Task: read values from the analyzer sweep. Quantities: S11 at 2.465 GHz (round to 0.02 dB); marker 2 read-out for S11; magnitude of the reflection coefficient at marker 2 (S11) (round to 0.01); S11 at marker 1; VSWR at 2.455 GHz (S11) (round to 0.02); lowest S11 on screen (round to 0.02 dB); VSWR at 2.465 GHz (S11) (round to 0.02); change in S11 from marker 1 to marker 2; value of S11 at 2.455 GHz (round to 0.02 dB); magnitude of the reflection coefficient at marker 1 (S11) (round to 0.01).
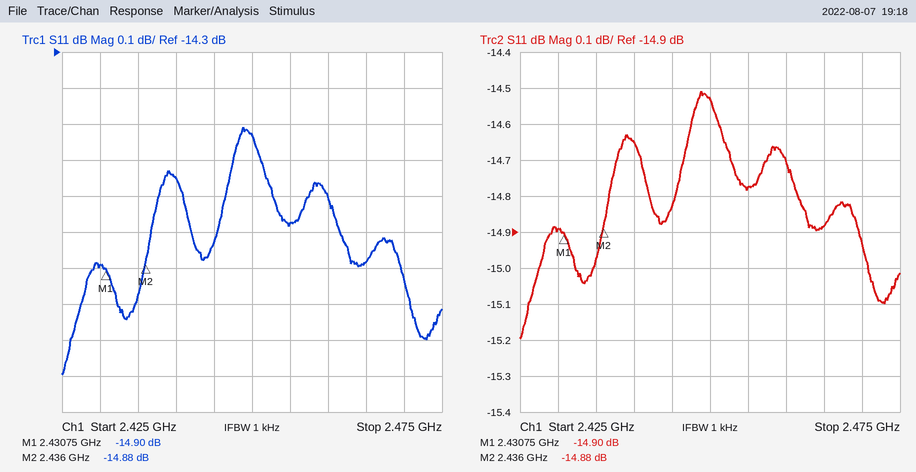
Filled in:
-14.88 dB
-14.88 dB
0.18
-14.90 dB
1.44
-15.20 dB
1.44
0.02 dB
-14.78 dB
0.18
